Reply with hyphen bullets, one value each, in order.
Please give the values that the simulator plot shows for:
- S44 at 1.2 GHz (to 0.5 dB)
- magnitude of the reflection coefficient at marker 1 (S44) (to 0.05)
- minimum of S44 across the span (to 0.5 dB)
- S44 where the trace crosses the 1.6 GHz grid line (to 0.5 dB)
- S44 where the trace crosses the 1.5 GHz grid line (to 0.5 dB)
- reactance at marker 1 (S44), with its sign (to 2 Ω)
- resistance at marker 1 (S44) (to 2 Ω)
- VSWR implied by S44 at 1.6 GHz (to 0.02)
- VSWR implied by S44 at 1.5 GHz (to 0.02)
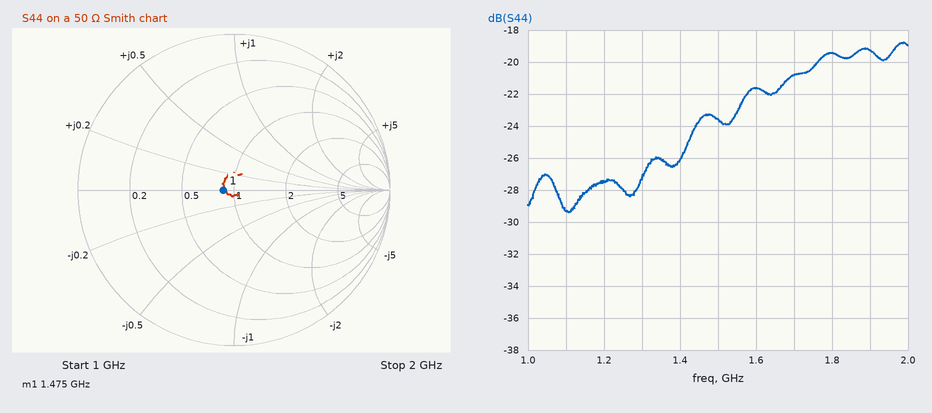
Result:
- -27.5 dB
- 0.05
- -29.5 dB
- -21.5 dB
- -23.5 dB
- 0 Ω
- 44 Ω
- 1.18
- 1.14
